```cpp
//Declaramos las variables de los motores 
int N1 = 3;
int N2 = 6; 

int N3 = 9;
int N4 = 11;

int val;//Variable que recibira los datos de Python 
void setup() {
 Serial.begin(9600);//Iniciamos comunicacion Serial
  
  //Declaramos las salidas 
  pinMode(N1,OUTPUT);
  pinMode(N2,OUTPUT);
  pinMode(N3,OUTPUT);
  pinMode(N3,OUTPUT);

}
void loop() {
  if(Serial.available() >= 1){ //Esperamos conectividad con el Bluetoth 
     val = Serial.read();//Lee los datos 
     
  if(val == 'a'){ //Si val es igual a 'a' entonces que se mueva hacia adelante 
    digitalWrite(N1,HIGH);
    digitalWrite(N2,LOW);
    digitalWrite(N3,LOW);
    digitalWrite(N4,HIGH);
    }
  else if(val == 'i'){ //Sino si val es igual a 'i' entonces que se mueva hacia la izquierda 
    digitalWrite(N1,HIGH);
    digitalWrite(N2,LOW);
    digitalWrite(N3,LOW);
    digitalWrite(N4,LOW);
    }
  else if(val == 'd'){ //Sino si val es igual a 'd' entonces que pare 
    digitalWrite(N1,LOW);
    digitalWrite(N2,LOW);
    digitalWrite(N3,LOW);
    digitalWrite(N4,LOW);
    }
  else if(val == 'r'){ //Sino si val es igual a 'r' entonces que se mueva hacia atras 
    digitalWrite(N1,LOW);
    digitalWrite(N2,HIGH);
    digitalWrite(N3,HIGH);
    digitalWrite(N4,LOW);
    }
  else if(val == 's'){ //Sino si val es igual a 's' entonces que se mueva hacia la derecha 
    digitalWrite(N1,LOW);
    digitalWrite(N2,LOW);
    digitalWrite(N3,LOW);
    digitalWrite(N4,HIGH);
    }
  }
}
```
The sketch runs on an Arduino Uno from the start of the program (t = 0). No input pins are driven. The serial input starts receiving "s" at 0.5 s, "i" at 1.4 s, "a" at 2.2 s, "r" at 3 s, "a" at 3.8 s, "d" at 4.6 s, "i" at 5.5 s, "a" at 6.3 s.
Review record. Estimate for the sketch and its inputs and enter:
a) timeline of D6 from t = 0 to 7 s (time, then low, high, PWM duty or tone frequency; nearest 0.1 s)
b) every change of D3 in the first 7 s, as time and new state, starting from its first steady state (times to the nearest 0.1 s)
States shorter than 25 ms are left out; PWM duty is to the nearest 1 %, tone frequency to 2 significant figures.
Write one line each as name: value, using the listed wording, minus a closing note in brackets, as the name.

timeline of D6 from t = 0 to 7 s: 0 s low; 3 s high; 3.8 s low
every change of D3 in the first 7 s, as time and new state, starting from its first steady state: 0 s low; 1.4 s high; 3 s low; 3.8 s high; 4.6 s low; 5.5 s high
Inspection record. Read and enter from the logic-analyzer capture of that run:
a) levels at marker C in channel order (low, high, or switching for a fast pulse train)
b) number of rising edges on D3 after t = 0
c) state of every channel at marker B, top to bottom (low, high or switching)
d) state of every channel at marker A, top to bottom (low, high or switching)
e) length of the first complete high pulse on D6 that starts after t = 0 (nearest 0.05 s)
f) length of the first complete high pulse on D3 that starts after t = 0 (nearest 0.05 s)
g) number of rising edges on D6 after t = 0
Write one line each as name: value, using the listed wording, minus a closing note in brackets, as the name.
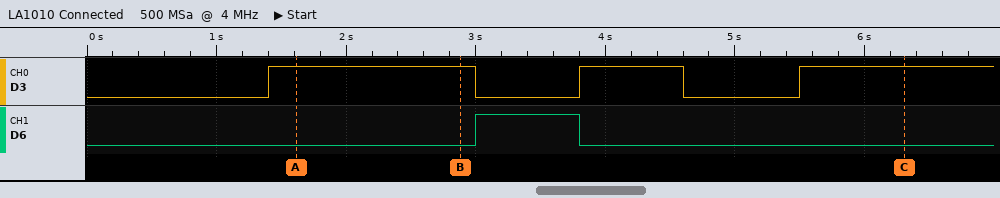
levels at marker C in channel order: D3 high, D6 low
number of rising edges on D3 after t = 0: 3
state of every channel at marker B, top to bottom: D3 high, D6 low
state of every channel at marker A, top to bottom: D3 high, D6 low
length of the first complete high pulse on D6 that starts after t = 0: 0.80 s
length of the first complete high pulse on D3 that starts after t = 0: 1.60 s
number of rising edges on D6 after t = 0: 1
